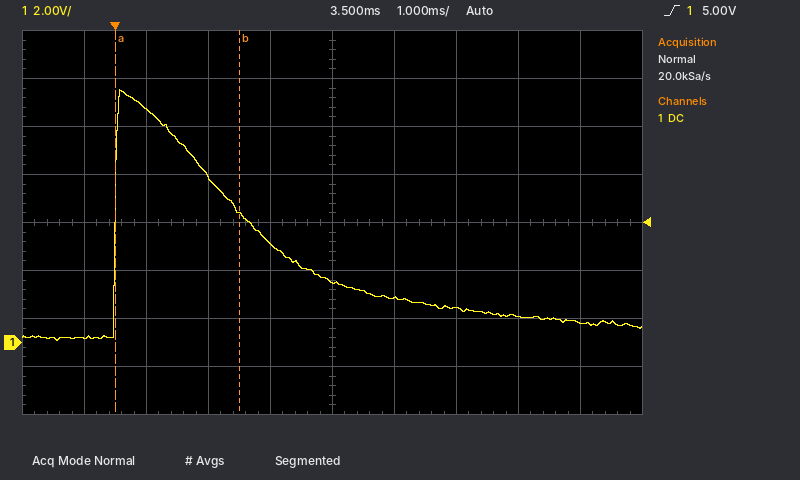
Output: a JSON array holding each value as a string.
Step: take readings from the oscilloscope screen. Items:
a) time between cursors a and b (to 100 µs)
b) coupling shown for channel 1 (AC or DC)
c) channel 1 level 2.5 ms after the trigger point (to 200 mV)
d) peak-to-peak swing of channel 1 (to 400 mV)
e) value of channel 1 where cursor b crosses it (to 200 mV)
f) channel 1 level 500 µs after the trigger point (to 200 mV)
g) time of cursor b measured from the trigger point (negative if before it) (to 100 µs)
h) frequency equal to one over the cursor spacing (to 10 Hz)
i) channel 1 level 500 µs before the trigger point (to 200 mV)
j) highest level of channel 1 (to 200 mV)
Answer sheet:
["2.0 ms", "DC", "4.2 V", "10.4 V", "5.4 V", "9.8 V", "+2.0 ms", "500 Hz", "200 mV", "10.6 V"]
